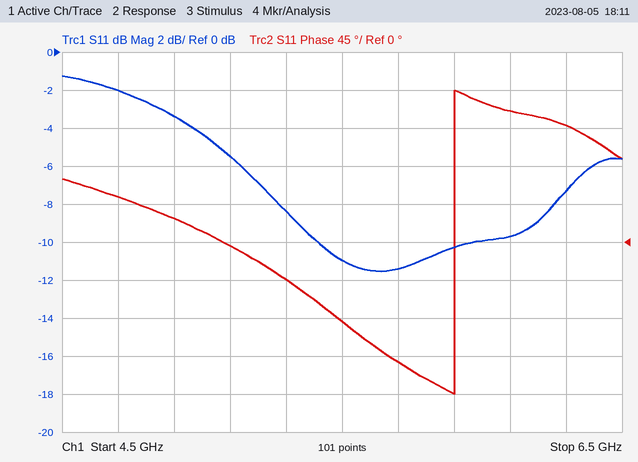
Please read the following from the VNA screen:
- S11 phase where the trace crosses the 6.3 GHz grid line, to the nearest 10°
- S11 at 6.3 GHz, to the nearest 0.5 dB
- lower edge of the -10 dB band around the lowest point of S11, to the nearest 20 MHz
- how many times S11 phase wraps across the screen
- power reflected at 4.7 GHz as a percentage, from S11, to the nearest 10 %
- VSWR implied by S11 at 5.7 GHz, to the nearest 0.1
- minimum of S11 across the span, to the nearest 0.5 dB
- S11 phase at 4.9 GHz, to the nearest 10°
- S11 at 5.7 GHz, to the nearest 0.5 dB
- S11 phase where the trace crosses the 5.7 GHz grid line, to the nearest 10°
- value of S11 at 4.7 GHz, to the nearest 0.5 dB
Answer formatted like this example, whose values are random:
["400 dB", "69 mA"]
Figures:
["140°", "-7.5 dB", "5.42 GHz", "1", "60 %", "1.7", "-11.5 dB", "30°", "-11.5 dB", "-140°", "-2.0 dB"]
